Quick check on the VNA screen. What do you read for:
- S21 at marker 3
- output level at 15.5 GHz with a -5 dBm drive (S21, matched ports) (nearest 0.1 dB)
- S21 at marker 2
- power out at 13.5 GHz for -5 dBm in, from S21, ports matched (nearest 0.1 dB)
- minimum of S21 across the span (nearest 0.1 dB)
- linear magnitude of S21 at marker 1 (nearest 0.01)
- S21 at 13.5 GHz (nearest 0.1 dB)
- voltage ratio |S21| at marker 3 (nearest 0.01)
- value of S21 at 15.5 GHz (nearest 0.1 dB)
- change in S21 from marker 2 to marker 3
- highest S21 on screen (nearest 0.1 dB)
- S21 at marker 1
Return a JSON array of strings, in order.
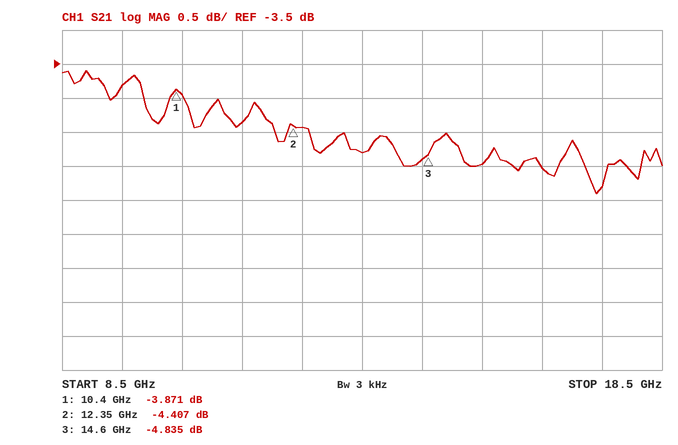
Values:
["-4.835 dB", "-10.0 dBm", "-4.407 dB", "-9.8 dBm", "-5.4 dB", "0.64", "-4.8 dB", "0.57", "-5.0 dB", "-0.428 dB", "-3.6 dB", "-3.871 dB"]
